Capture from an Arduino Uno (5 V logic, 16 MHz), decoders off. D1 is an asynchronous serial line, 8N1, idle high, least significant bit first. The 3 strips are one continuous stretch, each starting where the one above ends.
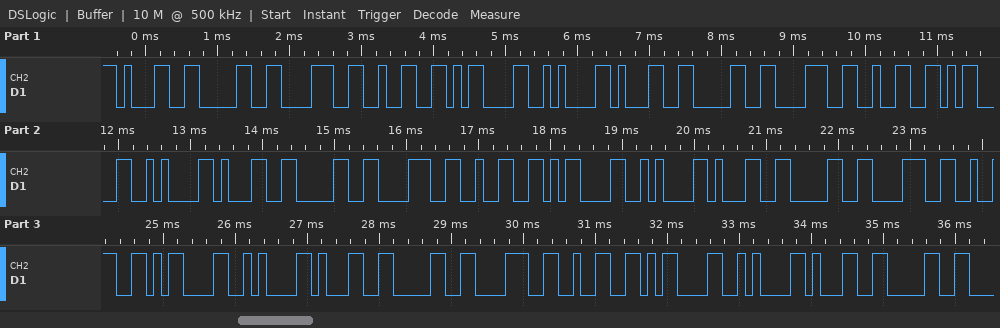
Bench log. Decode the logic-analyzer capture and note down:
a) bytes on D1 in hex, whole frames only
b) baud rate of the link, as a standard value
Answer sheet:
31 30 38 32 0D 0A 31 30 38 32 0D 0A 31 30 38 32 0D 0A 31 30 38 32 0D 0A 31 30 38 32 0D 0A 31 30
9600 baud
